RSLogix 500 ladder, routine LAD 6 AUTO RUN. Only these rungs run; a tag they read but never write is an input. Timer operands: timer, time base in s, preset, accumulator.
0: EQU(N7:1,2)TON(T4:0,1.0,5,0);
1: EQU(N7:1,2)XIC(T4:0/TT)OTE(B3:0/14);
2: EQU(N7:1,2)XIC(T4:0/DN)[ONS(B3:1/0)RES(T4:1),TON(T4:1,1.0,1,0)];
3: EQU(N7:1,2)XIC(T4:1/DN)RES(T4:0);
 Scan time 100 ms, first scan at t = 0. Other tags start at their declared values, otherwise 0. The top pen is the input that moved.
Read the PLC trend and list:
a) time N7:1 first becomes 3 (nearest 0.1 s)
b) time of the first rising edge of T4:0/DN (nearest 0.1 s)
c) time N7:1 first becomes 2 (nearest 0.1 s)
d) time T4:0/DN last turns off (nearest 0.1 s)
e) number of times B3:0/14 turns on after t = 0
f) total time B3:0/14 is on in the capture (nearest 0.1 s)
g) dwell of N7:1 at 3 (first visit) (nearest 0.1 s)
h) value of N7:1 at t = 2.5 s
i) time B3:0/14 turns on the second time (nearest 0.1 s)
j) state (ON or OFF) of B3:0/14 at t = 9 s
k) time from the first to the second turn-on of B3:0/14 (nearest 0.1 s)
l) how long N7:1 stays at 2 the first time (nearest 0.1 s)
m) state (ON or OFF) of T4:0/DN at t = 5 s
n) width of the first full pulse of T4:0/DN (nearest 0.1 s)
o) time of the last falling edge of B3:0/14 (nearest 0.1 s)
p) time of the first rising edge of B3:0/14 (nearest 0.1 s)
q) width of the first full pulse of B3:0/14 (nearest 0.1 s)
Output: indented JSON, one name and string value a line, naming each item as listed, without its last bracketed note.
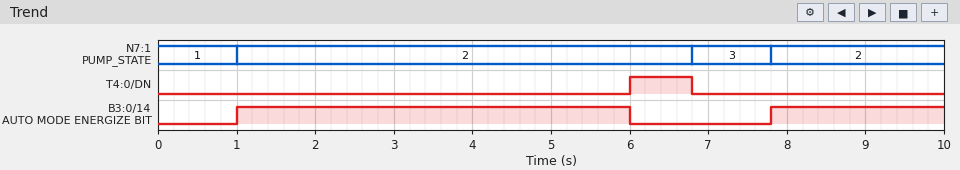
{
  "time N7:1 first becomes 3": "6.8 s",
  "time of the first rising edge of T4:0/DN": "6.0 s",
  "time N7:1 first becomes 2": "1.0 s",
  "time T4:0/DN last turns off": "6.8 s",
  "number of times B3:0/14 turns on after t = 0": "2",
  "total time B3:0/14 is on in the capture": "7.2 s",
  "dwell of N7:1 at 3 (first visit)": "1.0 s",
  "value of N7:1 at t = 2.5 s": "2",
  "time B3:0/14 turns on the second time": "7.8 s",
  "state (ON or OFF) of B3:0/14 at t = 9 s": "ON",
  "time from the first to the second turn-on of B3:0/14": "6.8 s",
  "how long N7:1 stays at 2 the first time": "5.8 s",
  "state (ON or OFF) of T4:0/DN at t = 5 s": "OFF",
  "width of the first full pulse of T4:0/DN": "0.8 s",
  "time of the last falling edge of B3:0/14": "6.0 s",
  "time of the first rising edge of B3:0/14": "1.0 s",
  "width of the first full pulse of B3:0/14": "5.0 s"
}
